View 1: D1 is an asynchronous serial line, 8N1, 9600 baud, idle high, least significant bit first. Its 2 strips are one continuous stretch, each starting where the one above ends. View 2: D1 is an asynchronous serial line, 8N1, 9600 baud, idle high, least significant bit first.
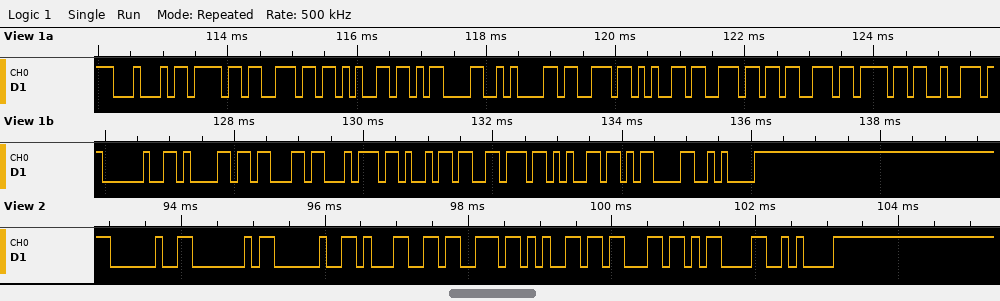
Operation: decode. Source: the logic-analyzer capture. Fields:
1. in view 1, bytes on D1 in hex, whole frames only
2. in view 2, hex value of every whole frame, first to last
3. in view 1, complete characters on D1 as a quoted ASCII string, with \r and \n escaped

44 6F 6E 65 0D 0A 73 65 6E 73 6F 72 20 61 63 74 69 76 65 0D 0A
20 40 20 31 73 65 63 0D 0A
"Done\r\nsensor active\r\n"
